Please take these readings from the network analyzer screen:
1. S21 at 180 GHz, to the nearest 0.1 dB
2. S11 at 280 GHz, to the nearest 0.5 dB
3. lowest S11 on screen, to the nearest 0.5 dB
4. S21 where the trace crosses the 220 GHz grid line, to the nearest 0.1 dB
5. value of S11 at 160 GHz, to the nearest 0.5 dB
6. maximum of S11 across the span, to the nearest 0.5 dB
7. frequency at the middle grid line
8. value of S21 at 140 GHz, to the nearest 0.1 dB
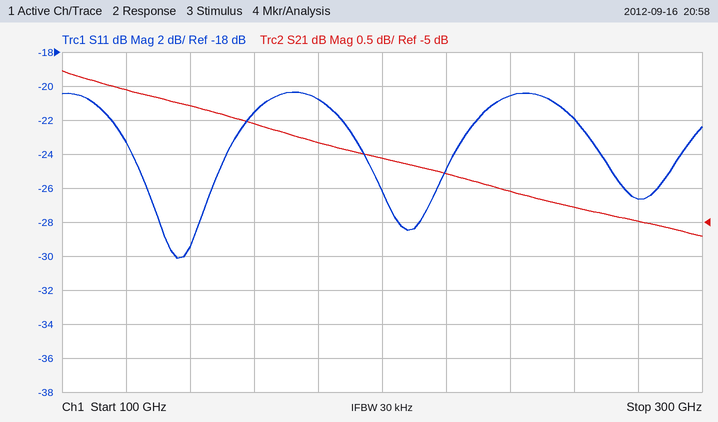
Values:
-3.8 dB
-26.5 dB
-30.0 dB
-4.3 dB
-21.5 dB
-20.5 dB
200 GHz
-3.3 dB
